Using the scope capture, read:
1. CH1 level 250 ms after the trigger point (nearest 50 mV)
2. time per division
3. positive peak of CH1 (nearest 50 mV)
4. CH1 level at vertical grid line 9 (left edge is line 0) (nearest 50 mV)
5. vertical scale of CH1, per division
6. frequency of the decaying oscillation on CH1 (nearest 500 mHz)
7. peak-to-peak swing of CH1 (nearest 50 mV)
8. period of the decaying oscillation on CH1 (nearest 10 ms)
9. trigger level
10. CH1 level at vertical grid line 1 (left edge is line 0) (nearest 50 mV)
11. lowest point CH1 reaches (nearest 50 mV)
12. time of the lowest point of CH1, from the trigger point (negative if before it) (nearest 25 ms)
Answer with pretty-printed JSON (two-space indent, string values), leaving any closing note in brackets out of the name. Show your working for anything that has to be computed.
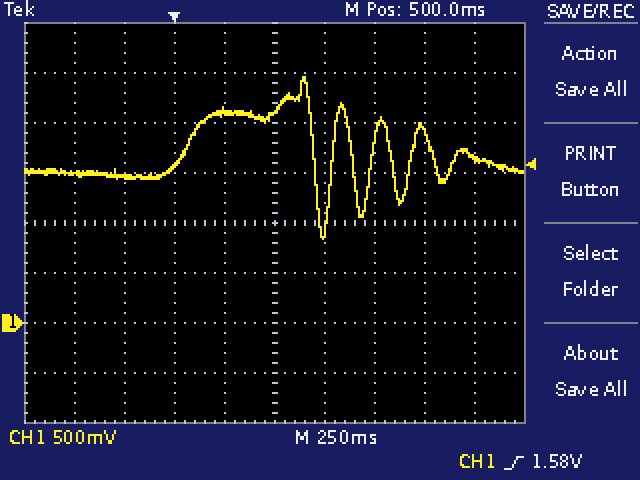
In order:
{
  "CH1 level 250 ms after the trigger point": "2.10 V",
  "time per division": "250 ms",
  "positive peak of CH1": "2.45 V",
  "CH1 level at vertical grid line 9 (left edge is line 0)": "1.65 V",
  "vertical scale of CH1, per division": "500 mV",
  "frequency of the decaying oscillation on CH1": "1 / 200 ms ≈ 5.0 Hz",
  "peak-to-peak swing of CH1": "2.45 V − (850 mV) = 1.60 V",
  "period of the decaying oscillation on CH1": "200 ms",
  "trigger level": "1.58 V",
  "CH1 level at vertical grid line 1 (left edge is line 0)": "1.50 V",
  "lowest point CH1 reaches": "850 mV",
  "time of the lowest point of CH1, from the trigger point (negative if before it)": "+750 ms"
}
